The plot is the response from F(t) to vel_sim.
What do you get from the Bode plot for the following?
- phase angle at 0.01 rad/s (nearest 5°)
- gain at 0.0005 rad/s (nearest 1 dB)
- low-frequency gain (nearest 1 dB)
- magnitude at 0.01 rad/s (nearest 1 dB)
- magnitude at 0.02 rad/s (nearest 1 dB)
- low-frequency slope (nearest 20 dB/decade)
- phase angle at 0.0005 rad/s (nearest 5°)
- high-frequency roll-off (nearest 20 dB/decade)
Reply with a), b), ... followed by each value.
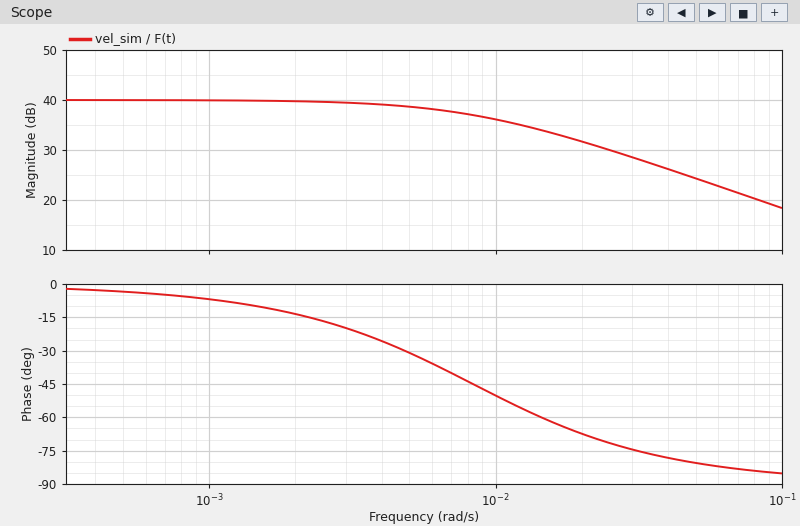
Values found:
a) -50°
b) 40 dB
c) 40 dB
d) 36 dB
e) 32 dB
f) 0 dB/decade
g) -5°
h) -20 dB/decade
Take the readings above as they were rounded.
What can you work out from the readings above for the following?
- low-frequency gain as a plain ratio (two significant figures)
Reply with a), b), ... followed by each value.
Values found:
a) 100
